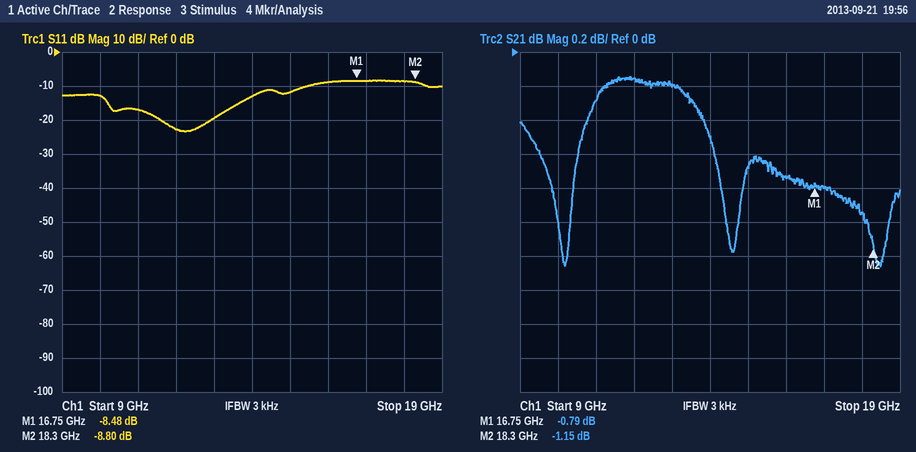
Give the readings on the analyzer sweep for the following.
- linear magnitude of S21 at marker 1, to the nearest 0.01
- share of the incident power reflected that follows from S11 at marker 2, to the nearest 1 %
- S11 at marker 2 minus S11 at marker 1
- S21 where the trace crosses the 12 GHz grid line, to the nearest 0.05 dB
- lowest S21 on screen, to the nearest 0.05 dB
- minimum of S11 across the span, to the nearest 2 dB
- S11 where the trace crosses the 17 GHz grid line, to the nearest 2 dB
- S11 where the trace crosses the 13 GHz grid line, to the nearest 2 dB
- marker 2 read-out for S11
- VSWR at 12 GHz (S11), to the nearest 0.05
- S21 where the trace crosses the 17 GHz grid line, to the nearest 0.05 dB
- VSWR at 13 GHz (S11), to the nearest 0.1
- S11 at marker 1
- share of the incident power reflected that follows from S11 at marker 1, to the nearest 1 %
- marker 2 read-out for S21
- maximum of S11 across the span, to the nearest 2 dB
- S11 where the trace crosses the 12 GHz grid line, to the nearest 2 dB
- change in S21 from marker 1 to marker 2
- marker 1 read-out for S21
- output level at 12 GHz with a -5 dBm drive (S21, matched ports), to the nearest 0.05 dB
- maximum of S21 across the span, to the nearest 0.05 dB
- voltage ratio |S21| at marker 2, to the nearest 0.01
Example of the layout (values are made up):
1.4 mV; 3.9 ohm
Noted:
0.91; 13 %; -0.32 dB; -0.15 dB; -1.25 dB; -24 dB; -8 dB; -20 dB; -8.80 dB; 1.15; -0.80 dB; 1.2; -8.48 dB; 14 %; -1.15 dB; -8 dB; -22 dB; -0.36 dB; -0.79 dB; -5.15 dBm; -0.15 dB; 0.88
